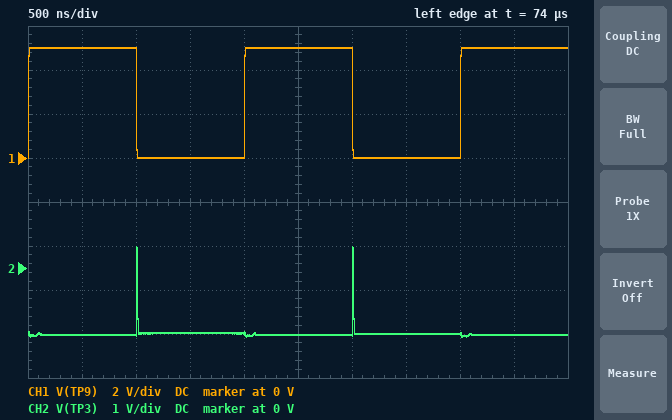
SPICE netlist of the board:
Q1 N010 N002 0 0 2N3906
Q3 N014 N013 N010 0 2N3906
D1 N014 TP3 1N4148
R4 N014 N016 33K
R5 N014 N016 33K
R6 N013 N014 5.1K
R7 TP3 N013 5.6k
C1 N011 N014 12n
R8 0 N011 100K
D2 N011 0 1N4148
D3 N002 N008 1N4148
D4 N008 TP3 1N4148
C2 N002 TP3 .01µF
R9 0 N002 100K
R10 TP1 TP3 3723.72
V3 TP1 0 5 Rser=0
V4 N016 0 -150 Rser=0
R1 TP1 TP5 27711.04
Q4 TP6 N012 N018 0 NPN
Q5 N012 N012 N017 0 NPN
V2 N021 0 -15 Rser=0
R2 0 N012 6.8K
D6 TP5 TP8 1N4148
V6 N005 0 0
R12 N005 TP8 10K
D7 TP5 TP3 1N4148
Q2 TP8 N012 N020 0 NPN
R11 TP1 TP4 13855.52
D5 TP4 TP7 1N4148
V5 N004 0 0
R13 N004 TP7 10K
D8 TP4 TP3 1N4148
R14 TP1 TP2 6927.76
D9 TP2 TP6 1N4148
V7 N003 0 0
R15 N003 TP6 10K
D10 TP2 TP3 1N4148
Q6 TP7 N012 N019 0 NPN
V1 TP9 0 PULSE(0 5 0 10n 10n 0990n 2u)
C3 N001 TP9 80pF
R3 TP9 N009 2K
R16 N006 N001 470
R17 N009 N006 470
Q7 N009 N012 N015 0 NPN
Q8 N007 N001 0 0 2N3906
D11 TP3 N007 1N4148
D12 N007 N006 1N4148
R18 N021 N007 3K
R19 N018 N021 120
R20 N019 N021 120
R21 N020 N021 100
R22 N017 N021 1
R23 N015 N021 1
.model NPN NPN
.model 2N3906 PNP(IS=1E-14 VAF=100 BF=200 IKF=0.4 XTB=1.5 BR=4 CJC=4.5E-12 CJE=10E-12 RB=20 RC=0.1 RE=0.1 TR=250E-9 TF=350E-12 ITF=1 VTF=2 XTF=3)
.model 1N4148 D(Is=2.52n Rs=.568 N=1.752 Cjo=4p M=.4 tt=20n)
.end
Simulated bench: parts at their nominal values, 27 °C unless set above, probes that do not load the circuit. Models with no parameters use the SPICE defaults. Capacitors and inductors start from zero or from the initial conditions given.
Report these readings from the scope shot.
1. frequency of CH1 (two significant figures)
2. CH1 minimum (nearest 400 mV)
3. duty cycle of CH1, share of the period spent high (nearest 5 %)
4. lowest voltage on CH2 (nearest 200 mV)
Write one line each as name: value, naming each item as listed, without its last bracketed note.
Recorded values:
frequency of CH1: 500 kHz
CH1 minimum: 0 V
duty cycle of CH1, share of the period spent high: 50 %
lowest voltage on CH2: -1.6 V
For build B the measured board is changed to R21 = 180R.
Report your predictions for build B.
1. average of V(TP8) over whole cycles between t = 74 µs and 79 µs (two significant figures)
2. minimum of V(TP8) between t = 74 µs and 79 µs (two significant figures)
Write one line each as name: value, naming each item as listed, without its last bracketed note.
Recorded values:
average of V(TP8) over whole cycles between t = 74 µs and 79 µs: -1.5 V
minimum of V(TP8) between t = 74 µs and 79 µs: -1.6 V
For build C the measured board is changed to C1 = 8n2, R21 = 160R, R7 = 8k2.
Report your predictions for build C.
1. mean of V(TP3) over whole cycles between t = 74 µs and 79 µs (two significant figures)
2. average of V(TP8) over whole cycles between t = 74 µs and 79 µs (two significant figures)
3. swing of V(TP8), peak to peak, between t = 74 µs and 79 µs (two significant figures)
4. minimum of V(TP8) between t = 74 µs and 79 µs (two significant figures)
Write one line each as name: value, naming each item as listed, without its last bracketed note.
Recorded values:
mean of V(TP3) over whole cycles between t = 74 µs and 79 µs: -1.5 V
average of V(TP8) over whole cycles between t = 74 µs and 79 µs: -1.6 V
swing of V(TP8), peak to peak, between t = 74 µs and 79 µs: 2.1 V
minimum of V(TP8) between t = 74 µs and 79 µs: -1.7 V
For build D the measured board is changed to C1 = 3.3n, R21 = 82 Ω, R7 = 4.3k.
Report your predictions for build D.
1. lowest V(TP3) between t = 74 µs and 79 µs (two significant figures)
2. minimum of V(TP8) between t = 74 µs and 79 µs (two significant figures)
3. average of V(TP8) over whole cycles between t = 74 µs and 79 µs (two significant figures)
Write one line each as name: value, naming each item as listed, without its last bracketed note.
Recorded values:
lowest V(TP3) between t = 74 µs and 79 µs: -1.5 V
minimum of V(TP8) between t = 74 µs and 79 µs: -2.9 V
average of V(TP8) over whole cycles between t = 74 µs and 79 µs: -2.3 V
